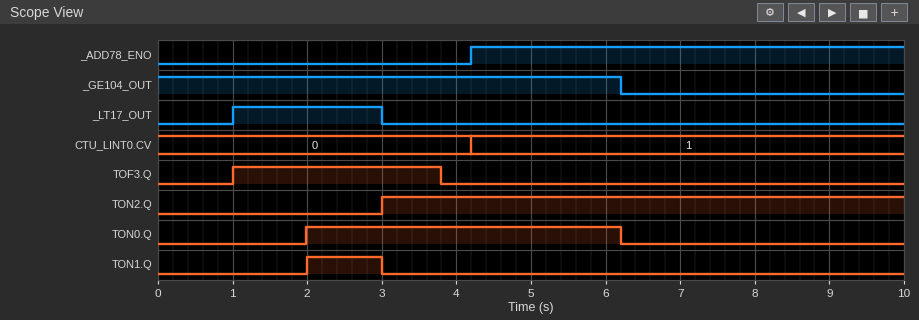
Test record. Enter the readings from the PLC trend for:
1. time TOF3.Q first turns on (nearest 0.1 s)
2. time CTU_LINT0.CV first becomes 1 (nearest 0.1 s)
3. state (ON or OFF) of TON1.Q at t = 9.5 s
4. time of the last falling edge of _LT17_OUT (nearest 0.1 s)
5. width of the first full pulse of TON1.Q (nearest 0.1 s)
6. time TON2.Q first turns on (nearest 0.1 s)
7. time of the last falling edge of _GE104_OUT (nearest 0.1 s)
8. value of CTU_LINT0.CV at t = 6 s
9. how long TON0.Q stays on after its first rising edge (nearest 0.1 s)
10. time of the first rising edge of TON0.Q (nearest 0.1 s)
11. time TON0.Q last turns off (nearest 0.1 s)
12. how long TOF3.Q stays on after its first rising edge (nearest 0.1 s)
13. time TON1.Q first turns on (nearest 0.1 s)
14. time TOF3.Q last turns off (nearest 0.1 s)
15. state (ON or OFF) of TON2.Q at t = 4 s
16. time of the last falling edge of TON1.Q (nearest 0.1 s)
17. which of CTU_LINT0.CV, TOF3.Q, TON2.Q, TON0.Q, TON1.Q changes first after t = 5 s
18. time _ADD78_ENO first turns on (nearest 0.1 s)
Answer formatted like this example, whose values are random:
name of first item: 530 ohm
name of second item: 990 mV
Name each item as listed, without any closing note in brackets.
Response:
time TOF3.Q first turns on: 1.0 s
time CTU_LINT0.CV first becomes 1: 4.2 s
state (ON or OFF) of TON1.Q at t = 9.5 s: OFF
time of the last falling edge of _LT17_OUT: 3.0 s
width of the first full pulse of TON1.Q: 1.0 s
time TON2.Q first turns on: 3.0 s
time of the last falling edge of _GE104_OUT: 6.2 s
value of CTU_LINT0.CV at t = 6 s: 1
how long TON0.Q stays on after its first rising edge: 4.2 s
time of the first rising edge of TON0.Q: 2.0 s
time TON0.Q last turns off: 6.2 s
how long TOF3.Q stays on after its first rising edge: 2.8 s
time TON1.Q first turns on: 2.0 s
time TOF3.Q last turns off: 3.8 s
state (ON or OFF) of TON2.Q at t = 4 s: ON
time of the last falling edge of TON1.Q: 3.0 s
which of CTU_LINT0.CV, TOF3.Q, TON2.Q, TON0.Q, TON1.Q changes first after t = 5 s: TON0.Q
time _ADD78_ENO first turns on: 4.2 s
